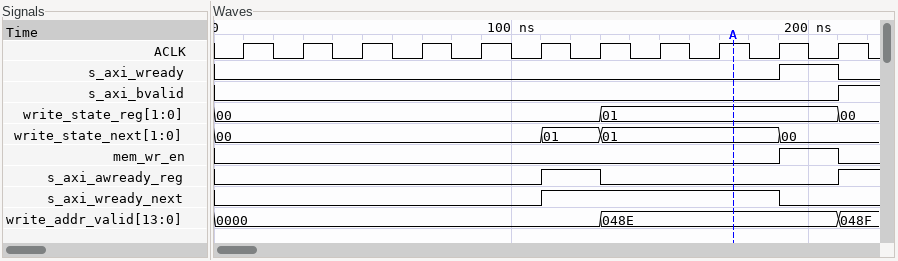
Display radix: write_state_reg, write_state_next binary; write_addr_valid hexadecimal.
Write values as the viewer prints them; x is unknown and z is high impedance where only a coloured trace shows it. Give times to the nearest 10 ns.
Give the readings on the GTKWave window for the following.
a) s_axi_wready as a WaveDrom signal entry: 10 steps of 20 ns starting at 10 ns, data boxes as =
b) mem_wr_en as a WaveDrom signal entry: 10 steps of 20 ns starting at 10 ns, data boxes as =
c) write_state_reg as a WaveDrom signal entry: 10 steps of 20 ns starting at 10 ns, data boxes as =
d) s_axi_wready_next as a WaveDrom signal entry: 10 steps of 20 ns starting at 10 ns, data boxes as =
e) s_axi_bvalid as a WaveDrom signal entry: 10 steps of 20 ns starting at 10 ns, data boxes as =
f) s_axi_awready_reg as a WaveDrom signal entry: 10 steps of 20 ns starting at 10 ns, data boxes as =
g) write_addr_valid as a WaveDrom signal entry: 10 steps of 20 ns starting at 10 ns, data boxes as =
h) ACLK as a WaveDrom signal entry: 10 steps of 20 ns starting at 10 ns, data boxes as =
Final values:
{name: 's_axi_wready', wave: '0........1'}
{name: 'mem_wr_en', wave: '0........1'}
{name: 'write_state_reg', wave: '=.....=...', data: '00 01'}
{name: 's_axi_wready_next', wave: '0....1...0'}
{name: 's_axi_bvalid', wave: '0.........'}
{name: 's_axi_awready_reg', wave: '0....10...'}
{name: 'write_addr_valid', wave: '=.....=...', data: '0000 048E'}
{name: 'ACLK', wave: 'p.........'}
